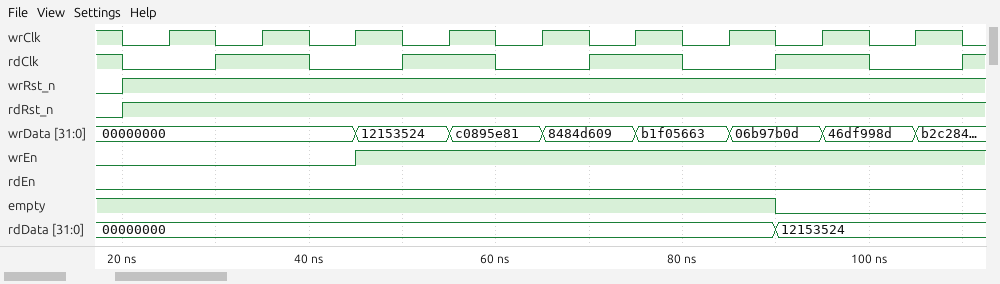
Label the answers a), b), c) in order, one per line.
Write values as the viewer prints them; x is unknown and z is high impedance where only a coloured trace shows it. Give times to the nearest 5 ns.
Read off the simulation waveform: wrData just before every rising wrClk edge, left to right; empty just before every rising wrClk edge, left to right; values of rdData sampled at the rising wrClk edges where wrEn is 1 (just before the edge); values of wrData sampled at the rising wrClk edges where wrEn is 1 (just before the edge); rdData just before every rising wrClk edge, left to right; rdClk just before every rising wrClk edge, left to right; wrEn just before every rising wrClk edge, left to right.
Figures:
a) 00000000, 00000000, 00000000, 12153524, c0895e81, 8484d609, b1f05663, 06b97b0d, 46df998d
b) 1 1 1 1 1 1 1 0 0
c) 00000000, 00000000, 00000000, 00000000, 12153524, 12153524
d) 12153524, c0895e81, 8484d609, b1f05663, 06b97b0d, 46df998d
e) 00000000, 00000000, 00000000, 00000000, 00000000, 00000000, 00000000, 12153524, 12153524
f) 0 1 0 1 0 1 0 1 0
g) 0 0 0 1 1 1 1 1 1
